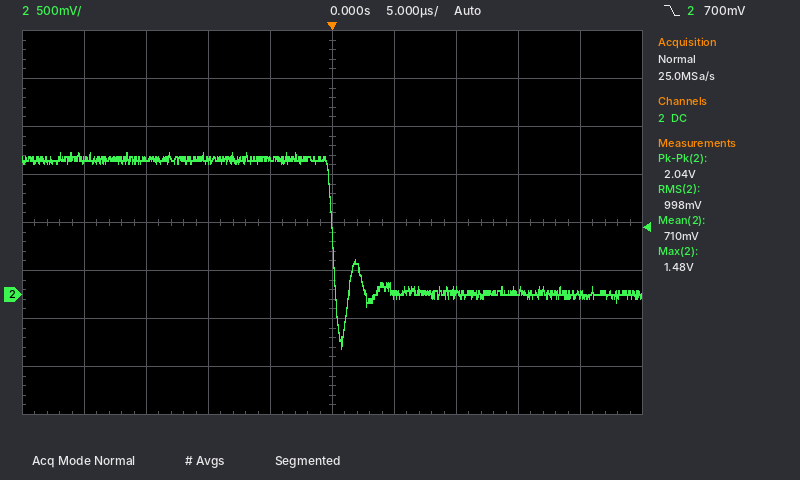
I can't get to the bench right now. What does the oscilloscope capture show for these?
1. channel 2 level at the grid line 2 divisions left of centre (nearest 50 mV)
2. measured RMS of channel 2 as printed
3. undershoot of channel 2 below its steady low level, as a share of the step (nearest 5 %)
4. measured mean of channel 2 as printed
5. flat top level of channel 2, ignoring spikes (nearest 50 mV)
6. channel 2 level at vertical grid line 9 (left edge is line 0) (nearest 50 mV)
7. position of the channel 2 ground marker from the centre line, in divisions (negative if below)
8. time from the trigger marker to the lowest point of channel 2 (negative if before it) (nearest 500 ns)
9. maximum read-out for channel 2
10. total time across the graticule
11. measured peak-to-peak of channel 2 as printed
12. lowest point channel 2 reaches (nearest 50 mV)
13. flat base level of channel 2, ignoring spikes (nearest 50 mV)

1.40 V
998 mV
40 %
710 mV
1.40 V
0 mV
-1.5 div
+1.0 µs
1.48 V
50 µs
2.04 V
-550 mV
0 mV
